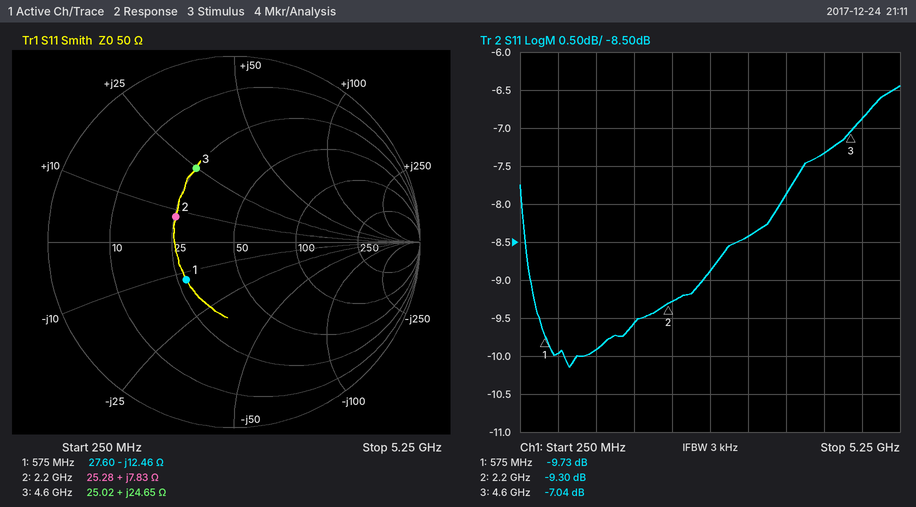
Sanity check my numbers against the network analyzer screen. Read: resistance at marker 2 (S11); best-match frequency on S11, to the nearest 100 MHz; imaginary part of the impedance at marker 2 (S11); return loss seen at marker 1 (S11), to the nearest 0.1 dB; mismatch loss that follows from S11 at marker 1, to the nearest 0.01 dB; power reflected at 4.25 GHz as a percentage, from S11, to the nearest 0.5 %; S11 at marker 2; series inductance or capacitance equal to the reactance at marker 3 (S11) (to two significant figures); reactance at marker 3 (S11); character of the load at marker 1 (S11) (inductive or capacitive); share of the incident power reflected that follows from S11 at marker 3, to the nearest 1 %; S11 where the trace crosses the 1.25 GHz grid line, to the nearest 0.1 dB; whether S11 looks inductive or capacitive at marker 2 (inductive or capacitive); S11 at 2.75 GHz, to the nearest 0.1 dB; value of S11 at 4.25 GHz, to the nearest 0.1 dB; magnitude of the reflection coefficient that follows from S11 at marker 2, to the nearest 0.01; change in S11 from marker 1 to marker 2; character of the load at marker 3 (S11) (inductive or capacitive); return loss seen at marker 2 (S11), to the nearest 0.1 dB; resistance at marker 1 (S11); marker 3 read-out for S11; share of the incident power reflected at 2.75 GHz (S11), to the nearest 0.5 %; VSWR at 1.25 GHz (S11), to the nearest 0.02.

25.28 Ω
900 MHz
+7.83 Ω
9.7 dB
0.49 dB
18.5 %
-9.30 dB
850 pH
+24.65 Ω
capacitive
20 %
-9.9 dB
inductive
-8.9 dB
-7.3 dB
0.34
0.43 dB
inductive
9.3 dB
27.60 Ω
-7.04 dB
13.0 %
1.94
